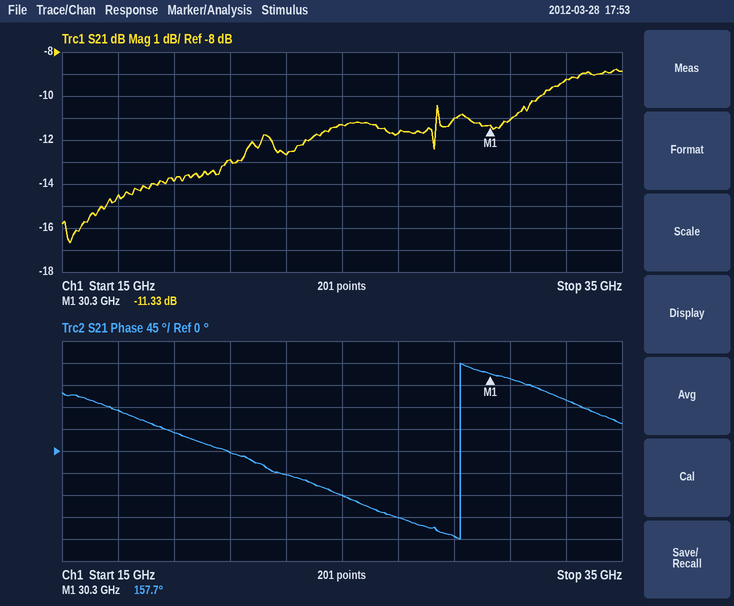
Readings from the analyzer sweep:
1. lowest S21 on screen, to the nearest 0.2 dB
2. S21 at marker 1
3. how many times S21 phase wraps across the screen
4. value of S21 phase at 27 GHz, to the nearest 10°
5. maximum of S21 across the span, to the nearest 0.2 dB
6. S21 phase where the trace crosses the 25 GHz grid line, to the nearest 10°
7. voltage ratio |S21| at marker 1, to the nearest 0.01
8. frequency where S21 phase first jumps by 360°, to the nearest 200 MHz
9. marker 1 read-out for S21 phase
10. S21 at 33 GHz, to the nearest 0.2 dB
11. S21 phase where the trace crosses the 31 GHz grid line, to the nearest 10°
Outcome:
-16.6 dB
-11.33 dB
1
-140°
-8.8 dB
-90°
0.27
29.2 GHz
157.7°
-9.2 dB
150°
